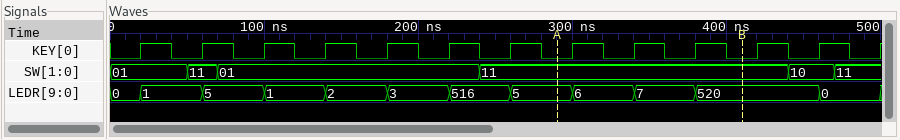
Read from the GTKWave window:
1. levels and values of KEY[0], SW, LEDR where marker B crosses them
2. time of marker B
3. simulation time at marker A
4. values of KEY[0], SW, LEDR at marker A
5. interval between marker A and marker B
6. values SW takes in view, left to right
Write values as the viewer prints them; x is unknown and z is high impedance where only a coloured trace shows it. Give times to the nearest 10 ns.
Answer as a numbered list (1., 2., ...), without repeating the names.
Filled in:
1. KEY[0]=0, SW=11, LEDR=520
2. 410 ns
3. 290 ns
4. KEY[0]=0, SW=11, LEDR=5
5. 120 ns
6. 01, 11, 01, 11, 10, 11
